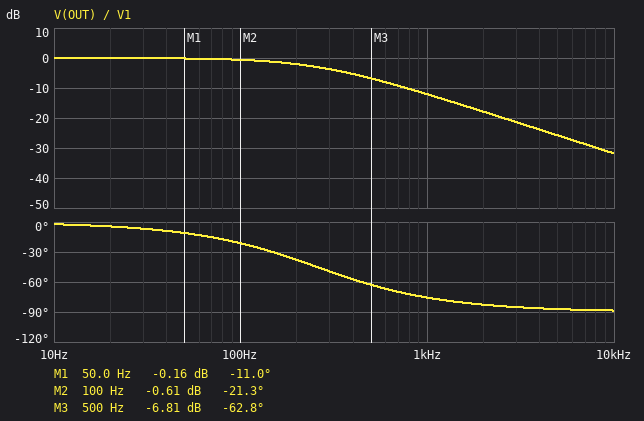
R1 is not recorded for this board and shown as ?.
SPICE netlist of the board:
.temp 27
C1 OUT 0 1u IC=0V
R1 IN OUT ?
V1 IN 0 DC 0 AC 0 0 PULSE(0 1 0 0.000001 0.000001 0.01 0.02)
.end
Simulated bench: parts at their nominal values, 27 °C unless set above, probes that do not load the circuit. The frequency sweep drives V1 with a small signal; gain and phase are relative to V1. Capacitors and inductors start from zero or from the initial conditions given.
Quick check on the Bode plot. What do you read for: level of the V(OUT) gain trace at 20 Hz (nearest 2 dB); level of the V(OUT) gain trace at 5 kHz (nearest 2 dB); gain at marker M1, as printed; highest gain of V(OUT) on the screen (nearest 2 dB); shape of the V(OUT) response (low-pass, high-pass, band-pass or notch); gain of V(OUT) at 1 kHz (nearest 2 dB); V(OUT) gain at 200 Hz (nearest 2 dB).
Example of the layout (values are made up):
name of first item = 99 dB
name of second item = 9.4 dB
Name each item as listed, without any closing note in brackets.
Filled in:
level of the V(OUT) gain trace at 20 Hz = 0 dB
level of the V(OUT) gain trace at 5 kHz = -26 dB
gain at marker M1, as printed = -0.16 dB
highest gain of V(OUT) on the screen = 0 dB
shape of the V(OUT) response = low-pass
gain of V(OUT) at 1 kHz = -12 dB
V(OUT) gain at 200 Hz = -2 dB
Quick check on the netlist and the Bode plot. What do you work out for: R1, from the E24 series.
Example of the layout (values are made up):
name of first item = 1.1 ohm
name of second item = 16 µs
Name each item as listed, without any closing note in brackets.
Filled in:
R1, from the E24 series = 620 Ω
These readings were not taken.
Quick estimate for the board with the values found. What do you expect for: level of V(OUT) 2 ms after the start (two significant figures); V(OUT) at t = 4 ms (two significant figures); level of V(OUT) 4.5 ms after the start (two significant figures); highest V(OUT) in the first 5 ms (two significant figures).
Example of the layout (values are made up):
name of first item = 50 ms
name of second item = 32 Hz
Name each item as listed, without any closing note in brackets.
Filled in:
level of V(OUT) 2 ms after the start = 960 mV
V(OUT) at t = 4 ms = 1.0 V
level of V(OUT) 4.5 ms after the start = 1.0 V
highest V(OUT) in the first 5 ms = 1.0 V
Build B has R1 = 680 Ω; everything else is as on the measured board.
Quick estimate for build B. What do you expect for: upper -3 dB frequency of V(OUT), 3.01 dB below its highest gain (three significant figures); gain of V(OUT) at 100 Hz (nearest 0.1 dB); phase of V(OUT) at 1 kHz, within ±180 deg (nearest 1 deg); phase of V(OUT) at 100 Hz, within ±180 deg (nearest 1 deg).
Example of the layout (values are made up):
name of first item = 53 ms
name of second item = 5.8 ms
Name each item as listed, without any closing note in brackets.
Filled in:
upper -3 dB frequency of V(OUT), 3.01 dB below its highest gain = 234 Hz
gain of V(OUT) at 100 Hz = -0.7 dB
phase of V(OUT) at 1 kHz, within ±180 deg = -77 deg
phase of V(OUT) at 100 Hz, within ±180 deg = -23 deg
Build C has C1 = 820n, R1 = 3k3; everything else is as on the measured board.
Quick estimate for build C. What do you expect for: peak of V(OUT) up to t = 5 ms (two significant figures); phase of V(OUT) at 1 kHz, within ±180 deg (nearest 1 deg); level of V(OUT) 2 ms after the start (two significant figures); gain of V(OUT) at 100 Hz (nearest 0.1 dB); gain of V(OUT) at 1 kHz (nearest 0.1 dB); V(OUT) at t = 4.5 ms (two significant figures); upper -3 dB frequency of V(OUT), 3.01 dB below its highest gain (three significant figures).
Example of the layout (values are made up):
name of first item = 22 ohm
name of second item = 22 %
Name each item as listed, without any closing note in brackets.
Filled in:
peak of V(OUT) up to t = 5 ms = 840 mV
phase of V(OUT) at 1 kHz, within ±180 deg = -87 deg
level of V(OUT) 2 ms after the start = 520 mV
gain of V(OUT) at 100 Hz = -5.9 dB
gain of V(OUT) at 1 kHz = -24.6 dB
V(OUT) at t = 4.5 ms = 810 mV
upper -3 dB frequency of V(OUT), 3.01 dB below its highest gain = 58.8 Hz
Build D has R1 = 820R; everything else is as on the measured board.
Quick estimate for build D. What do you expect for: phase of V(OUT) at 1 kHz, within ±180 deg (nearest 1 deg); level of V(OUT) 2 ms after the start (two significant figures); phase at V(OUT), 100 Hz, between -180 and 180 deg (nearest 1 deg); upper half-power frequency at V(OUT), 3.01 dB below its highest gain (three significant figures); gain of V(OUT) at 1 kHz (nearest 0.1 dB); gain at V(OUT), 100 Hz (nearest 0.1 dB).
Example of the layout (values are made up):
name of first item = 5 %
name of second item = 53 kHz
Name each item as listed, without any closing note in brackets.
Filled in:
phase of V(OUT) at 1 kHz, within ±180 deg = -79 deg
level of V(OUT) 2 ms after the start = 910 mV
phase at V(OUT), 100 Hz, between -180 and 180 deg = -27 deg
upper half-power frequency at V(OUT), 3.01 dB below its highest gain = 194 Hz
gain of V(OUT) at 1 kHz = -14.4 dB
gain at V(OUT), 100 Hz = -1.0 dB
